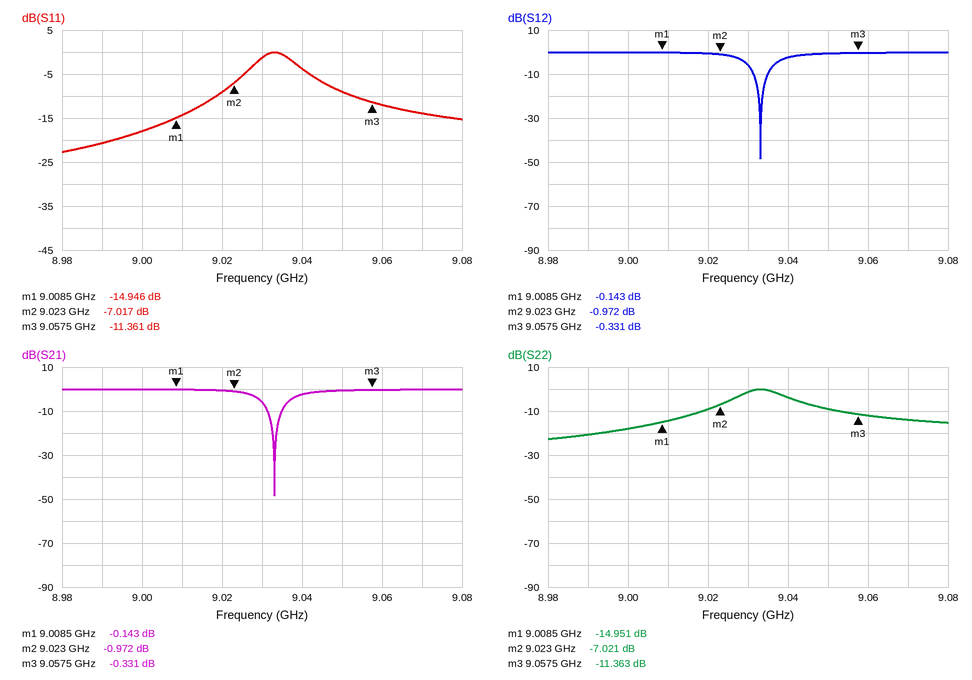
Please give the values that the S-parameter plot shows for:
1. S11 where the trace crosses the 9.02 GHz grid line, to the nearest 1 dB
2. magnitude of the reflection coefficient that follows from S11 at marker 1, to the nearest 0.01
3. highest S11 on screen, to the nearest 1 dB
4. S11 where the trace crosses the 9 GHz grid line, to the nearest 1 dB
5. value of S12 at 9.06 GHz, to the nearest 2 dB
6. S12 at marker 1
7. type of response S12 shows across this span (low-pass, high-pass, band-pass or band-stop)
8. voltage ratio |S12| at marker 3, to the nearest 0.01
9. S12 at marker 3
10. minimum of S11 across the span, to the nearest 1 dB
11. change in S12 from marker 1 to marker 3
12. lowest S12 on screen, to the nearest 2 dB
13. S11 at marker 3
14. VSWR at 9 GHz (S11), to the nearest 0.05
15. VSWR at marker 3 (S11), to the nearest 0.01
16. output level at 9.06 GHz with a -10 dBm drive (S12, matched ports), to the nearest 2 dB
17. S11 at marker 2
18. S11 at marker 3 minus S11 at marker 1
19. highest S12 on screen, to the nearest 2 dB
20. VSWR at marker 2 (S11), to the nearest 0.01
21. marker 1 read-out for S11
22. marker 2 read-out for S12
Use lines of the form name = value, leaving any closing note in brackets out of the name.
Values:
S11 where the trace crosses the 9.02 GHz grid line, to the nearest 1 dB = -9 dB
magnitude of the reflection coefficient that follows from S11 at marker 1, to the nearest 0.01 = 0.18
highest S11 on screen, to the nearest 1 dB = 0 dB
S11 where the trace crosses the 9 GHz grid line, to the nearest 1 dB = -18 dB
value of S12 at 9.06 GHz, to the nearest 2 dB = 0 dB
S12 at marker 1 = -0.143 dB
type of response S12 shows across this span = band-stop
voltage ratio |S12| at marker 3, to the nearest 0.01 = 0.96
S12 at marker 3 = -0.331 dB
minimum of S11 across the span, to the nearest 1 dB = -23 dB
change in S12 from marker 1 to marker 3 = -0.188 dB
lowest S12 on screen, to the nearest 2 dB = -48 dB
S11 at marker 3 = -11.361 dB
VSWR at 9 GHz (S11), to the nearest 0.05 = 1.30
VSWR at marker 3 (S11), to the nearest 0.01 = 1.74
output level at 9.06 GHz with a -10 dBm drive (S12, matched ports), to the nearest 2 dB = -10 dBm
S11 at marker 2 = -7.017 dB
S11 at marker 3 minus S11 at marker 1 = 3.585 dB
highest S12 on screen, to the nearest 2 dB = 0 dB
VSWR at marker 2 (S11), to the nearest 0.01 = 2.61
marker 1 read-out for S11 = -14.946 dB
marker 2 read-out for S12 = -0.972 dB
